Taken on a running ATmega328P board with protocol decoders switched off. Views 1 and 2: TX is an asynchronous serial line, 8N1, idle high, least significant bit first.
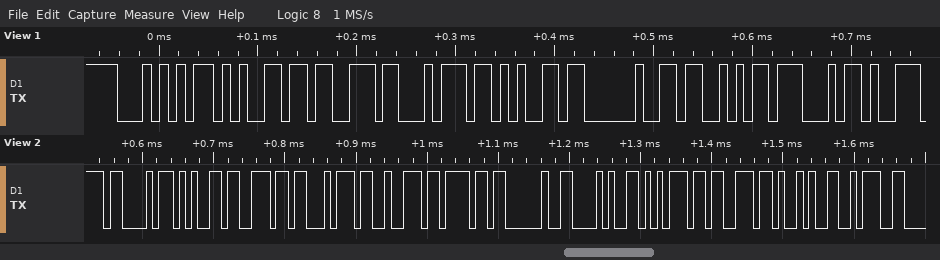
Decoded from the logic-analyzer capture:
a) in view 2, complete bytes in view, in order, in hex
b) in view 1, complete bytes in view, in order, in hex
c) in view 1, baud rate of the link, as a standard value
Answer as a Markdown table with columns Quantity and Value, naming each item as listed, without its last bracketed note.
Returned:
| Quantity | Value |
|---|---|
| in view 2, complete bytes in view, in order, in hex | 0x43 0x65 0x6E 0x74 0x72 0x6F 0x20 0x28 0x75 0x73 0x29 0x3A |
| in view 1, complete bytes in view, in order, in hex | 54 65 73 74 65 20 53 47 |
| in view 1, baud rate of the link, as a standard value | 115200 baud |
